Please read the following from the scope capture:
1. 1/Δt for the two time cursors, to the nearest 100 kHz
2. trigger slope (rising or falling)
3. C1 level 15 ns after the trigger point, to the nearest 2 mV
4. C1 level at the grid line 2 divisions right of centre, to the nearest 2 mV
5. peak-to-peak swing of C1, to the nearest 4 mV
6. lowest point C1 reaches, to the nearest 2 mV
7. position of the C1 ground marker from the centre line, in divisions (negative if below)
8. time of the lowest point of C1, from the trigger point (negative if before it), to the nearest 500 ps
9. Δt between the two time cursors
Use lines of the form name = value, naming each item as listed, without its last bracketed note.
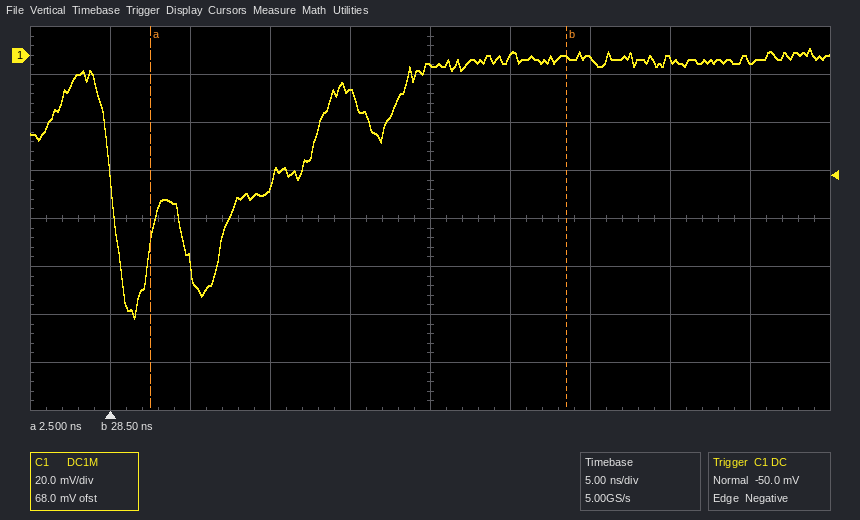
1/Δt for the two time cursors, to the nearest 100 kHz = 38.5 MHz
trigger slope = falling
C1 level 15 ns after the trigger point, to the nearest 2 mV = -16 mV
C1 level at the grid line 2 divisions right of centre, to the nearest 2 mV = -2 mV
peak-to-peak swing of C1, to the nearest 4 mV = 112 mV
lowest point C1 reaches, to the nearest 2 mV = -110 mV
position of the C1 ground marker from the centre line, in divisions = +3.4 div
time of the lowest point of C1, from the trigger point (negative if before it), to the nearest 500 ps = +1.5 ns
Δt between the two time cursors = 26.0 ns
